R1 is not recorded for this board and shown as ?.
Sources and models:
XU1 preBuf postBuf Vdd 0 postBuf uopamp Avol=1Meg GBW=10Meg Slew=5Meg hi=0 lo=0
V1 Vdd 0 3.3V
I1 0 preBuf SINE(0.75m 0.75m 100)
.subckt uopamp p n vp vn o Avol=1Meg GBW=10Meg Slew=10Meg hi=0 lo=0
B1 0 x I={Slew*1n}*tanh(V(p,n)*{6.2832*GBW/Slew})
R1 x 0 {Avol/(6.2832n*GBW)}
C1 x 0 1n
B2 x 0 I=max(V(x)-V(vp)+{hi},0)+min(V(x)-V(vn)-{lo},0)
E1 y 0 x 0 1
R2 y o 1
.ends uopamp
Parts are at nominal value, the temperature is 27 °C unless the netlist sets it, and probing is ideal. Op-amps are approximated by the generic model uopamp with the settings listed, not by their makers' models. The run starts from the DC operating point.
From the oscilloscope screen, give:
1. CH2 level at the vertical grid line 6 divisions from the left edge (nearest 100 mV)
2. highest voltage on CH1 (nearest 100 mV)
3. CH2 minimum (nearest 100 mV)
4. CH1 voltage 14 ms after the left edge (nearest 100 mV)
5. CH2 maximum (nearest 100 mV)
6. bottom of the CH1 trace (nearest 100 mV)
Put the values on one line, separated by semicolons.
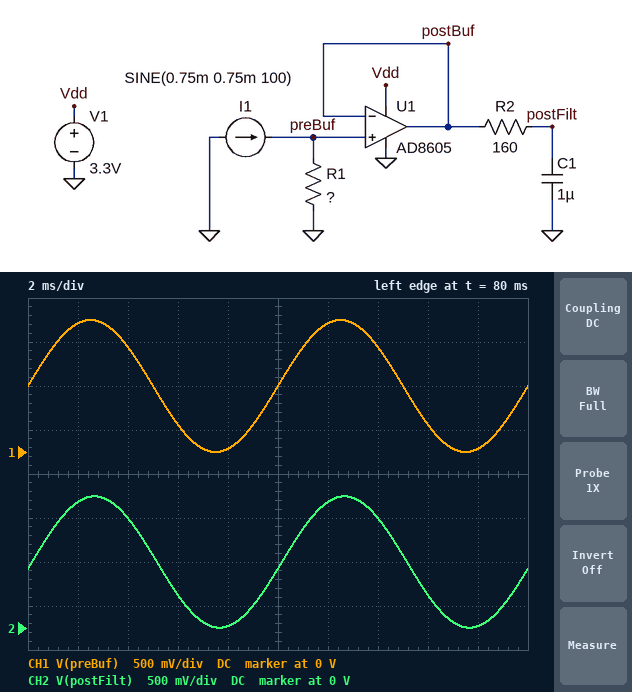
1.4 V; 1.5 V; 0 V; 1.2 V; 1.5 V; 0 V
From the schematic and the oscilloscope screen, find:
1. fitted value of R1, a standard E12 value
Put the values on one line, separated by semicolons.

1 kΩ
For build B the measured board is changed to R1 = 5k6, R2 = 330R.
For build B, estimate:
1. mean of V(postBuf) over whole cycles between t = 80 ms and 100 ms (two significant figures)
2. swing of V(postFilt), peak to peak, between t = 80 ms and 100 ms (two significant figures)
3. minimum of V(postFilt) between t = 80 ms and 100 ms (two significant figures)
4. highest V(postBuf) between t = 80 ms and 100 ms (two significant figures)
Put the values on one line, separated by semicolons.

2.4 V; 3.2 V; 87 mV; 3.3 V
